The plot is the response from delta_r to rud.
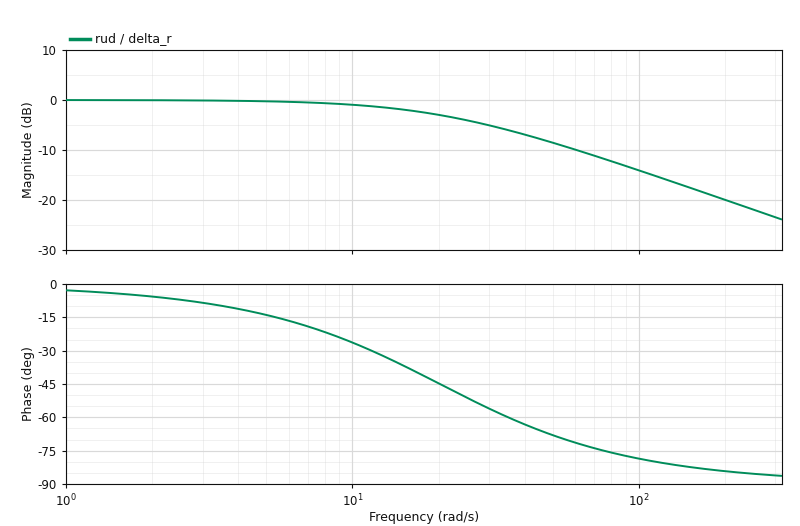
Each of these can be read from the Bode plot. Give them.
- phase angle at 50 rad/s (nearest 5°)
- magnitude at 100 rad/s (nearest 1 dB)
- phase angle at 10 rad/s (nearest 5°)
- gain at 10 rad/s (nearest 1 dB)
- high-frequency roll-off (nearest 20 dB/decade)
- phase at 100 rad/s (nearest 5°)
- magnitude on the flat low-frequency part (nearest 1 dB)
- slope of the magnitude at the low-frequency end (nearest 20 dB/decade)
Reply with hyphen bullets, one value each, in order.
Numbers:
- -70°
- -14 dB
- -25°
- -1 dB
- -20 dB/decade
- -80°
- 0 dB
- 0 dB/decade
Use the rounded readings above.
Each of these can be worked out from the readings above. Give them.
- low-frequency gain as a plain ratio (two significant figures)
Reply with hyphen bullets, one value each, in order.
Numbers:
- 1.0
